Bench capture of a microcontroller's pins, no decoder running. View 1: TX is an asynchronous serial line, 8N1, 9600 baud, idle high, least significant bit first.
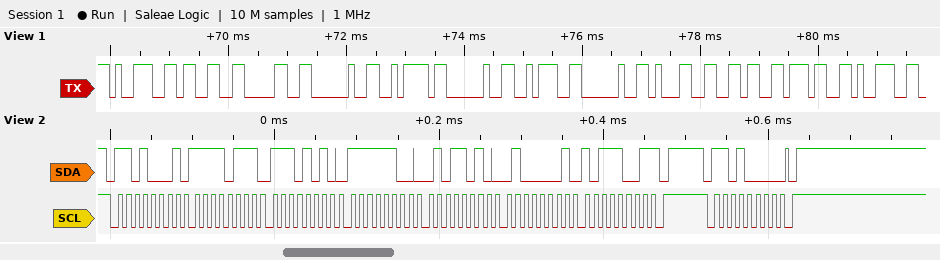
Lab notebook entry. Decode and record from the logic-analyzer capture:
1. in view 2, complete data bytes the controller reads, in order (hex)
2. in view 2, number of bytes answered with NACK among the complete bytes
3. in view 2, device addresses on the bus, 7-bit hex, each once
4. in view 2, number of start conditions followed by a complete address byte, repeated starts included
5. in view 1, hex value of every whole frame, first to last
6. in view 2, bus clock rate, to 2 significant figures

F7 EA FC 5A 41 B9
1
0x68
2
0x39 0x33 0x30 0x20 0x7A 0x20 0x3A 0x20 0x31 0x36 0x37 0x39
100 kHz
